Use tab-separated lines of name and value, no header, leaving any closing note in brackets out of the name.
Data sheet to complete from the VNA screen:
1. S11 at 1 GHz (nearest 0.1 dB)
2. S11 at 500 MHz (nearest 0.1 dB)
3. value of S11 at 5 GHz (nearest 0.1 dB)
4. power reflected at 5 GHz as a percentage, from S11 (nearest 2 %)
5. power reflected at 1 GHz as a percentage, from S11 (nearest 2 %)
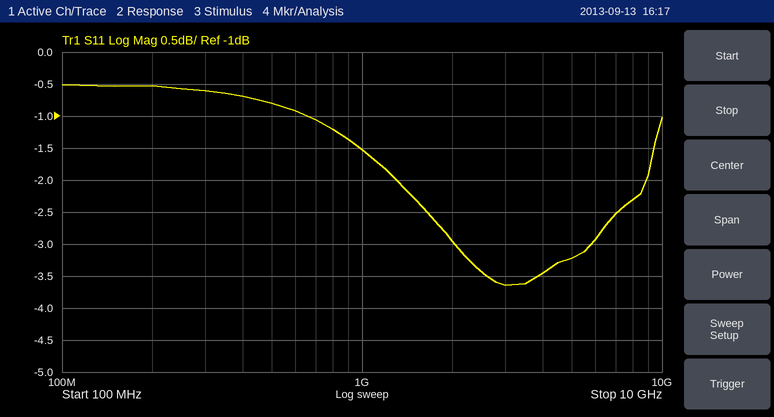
S11 at 1 GHz	-1.5 dB
S11 at 500 MHz	-0.8 dB
value of S11 at 5 GHz	-3.2 dB
power reflected at 5 GHz as a percentage, from S11	48 %
power reflected at 1 GHz as a percentage, from S11	70 %
